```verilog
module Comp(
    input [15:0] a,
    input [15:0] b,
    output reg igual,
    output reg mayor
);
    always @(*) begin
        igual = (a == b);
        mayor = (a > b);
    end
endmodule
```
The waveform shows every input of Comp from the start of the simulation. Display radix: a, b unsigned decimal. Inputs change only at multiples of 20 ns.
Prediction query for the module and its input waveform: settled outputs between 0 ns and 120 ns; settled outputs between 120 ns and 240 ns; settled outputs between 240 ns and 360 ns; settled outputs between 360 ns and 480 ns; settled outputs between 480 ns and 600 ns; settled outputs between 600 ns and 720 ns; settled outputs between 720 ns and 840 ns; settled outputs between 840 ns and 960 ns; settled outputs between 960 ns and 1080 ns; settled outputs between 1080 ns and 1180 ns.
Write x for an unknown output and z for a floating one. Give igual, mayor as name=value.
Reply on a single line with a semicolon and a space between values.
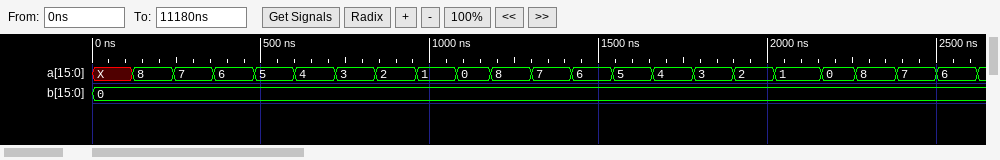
igual=x, mayor=x; igual=0, mayor=1; igual=0, mayor=1; igual=0, mayor=1; igual=0, mayor=1; igual=0, mayor=1; igual=0, mayor=1; igual=0, mayor=1; igual=0, mayor=1; igual=1, mayor=0
